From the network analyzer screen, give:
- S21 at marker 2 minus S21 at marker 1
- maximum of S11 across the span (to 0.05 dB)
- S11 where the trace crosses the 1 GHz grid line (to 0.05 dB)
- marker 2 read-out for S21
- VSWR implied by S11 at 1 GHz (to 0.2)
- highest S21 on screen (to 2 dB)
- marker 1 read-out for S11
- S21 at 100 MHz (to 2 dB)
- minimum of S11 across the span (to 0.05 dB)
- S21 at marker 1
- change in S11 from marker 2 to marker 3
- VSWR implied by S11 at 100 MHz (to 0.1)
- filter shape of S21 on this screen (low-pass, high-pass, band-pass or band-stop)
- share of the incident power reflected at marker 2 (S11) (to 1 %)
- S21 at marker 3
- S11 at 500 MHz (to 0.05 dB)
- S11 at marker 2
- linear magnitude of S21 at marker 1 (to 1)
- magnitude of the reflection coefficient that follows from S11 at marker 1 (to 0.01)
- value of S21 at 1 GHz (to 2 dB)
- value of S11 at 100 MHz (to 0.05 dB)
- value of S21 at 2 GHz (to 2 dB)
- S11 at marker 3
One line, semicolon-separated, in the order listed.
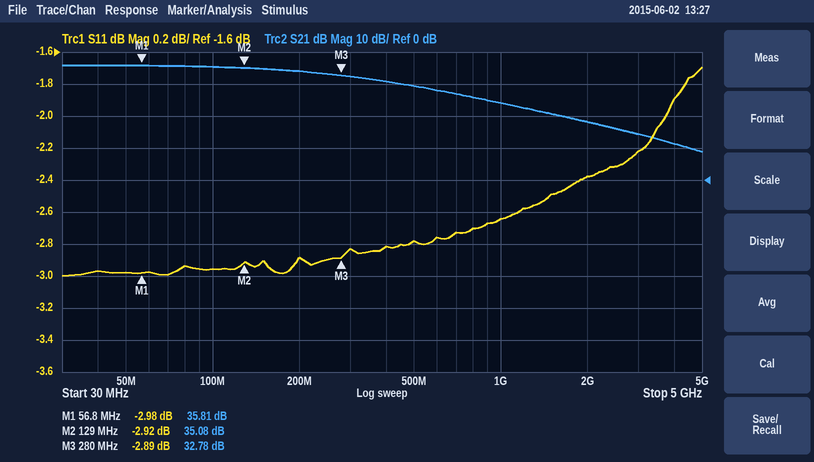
-0.73 dB; -1.70 dB; -2.65 dB; 35.08 dB; 6.6; 36 dB; -2.98 dB; 36 dB; -3.00 dB; 35.81 dB; 0.03 dB; 5.9; low-pass; 51 %; 32.78 dB; -2.80 dB; -2.92 dB; 62; 0.71; 24 dB; -2.95 dB; 18 dB; -2.89 dB
